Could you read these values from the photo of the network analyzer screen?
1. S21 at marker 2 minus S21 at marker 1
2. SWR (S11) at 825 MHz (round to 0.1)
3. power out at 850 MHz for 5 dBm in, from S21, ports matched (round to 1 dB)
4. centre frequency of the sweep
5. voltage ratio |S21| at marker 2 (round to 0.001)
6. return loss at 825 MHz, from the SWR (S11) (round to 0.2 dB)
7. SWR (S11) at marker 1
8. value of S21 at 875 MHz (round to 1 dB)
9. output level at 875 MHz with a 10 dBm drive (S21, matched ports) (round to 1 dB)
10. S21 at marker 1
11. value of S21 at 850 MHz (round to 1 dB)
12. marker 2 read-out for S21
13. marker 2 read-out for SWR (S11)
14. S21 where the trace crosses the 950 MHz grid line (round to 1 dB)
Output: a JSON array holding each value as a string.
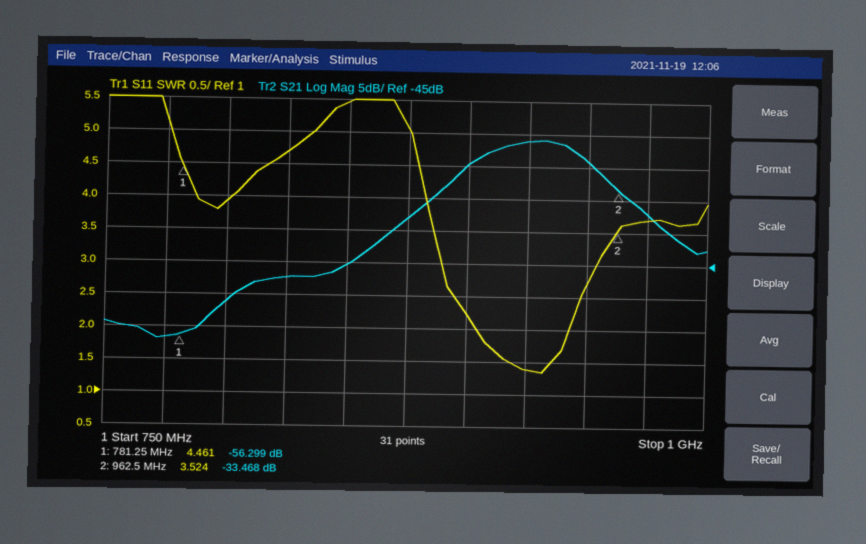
["22.831 dB", "4.7", "-40 dBm", "875 MHz", "0.021", "3.8 dB", "4.461", "-38 dB", "-28 dBm", "-56.299 dB", "-45 dB", "-33.468 dB", "3.524", "-29 dB"]
